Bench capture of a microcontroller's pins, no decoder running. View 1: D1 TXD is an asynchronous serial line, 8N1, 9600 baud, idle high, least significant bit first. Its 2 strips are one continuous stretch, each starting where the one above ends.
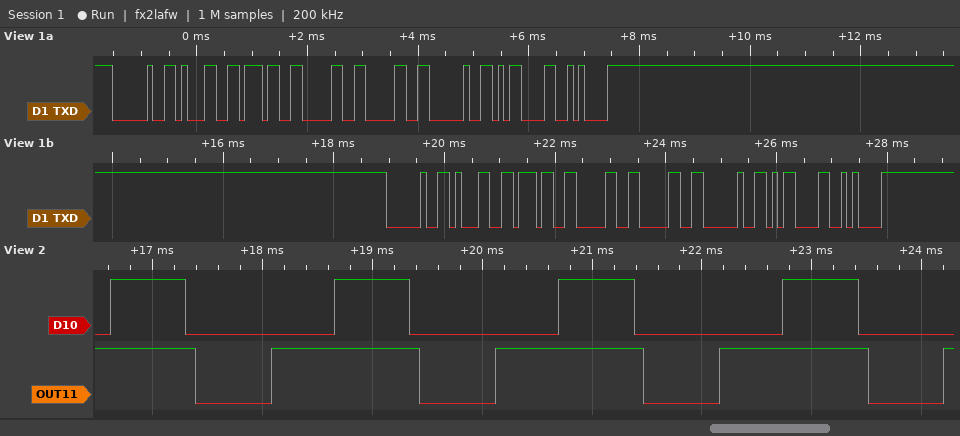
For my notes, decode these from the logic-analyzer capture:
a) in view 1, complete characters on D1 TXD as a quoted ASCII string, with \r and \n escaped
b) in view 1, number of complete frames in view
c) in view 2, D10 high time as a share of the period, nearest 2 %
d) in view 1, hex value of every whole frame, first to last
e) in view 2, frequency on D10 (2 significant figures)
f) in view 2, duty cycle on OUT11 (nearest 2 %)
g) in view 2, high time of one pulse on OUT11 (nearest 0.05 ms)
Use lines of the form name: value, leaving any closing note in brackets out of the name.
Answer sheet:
in view 1, complete characters on D1 TXD as a quoted ASCII string, with \r and \n escaped: " 1700 \r\n 1700 \r\n"
in view 1, number of complete frames in view: 16
in view 2, D10 high time as a share of the period, nearest 2 %: 34 %
in view 1, hex value of every whole frame, first to last: 20 31 37 30 30 20 0D 0A 20 31 37 30 30 20 0D 0A
in view 2, frequency on D10: 490 Hz
in view 2, duty cycle on OUT11: 66 %
in view 2, high time of one pulse on OUT11: 1.35 ms
